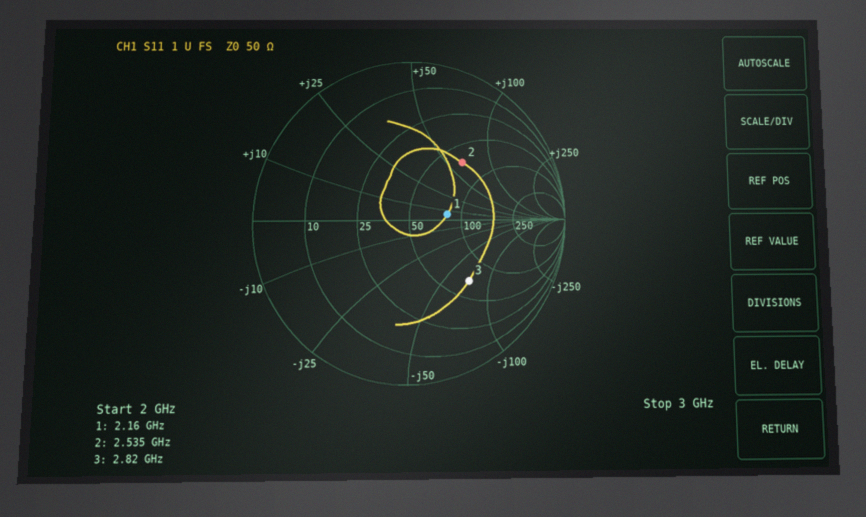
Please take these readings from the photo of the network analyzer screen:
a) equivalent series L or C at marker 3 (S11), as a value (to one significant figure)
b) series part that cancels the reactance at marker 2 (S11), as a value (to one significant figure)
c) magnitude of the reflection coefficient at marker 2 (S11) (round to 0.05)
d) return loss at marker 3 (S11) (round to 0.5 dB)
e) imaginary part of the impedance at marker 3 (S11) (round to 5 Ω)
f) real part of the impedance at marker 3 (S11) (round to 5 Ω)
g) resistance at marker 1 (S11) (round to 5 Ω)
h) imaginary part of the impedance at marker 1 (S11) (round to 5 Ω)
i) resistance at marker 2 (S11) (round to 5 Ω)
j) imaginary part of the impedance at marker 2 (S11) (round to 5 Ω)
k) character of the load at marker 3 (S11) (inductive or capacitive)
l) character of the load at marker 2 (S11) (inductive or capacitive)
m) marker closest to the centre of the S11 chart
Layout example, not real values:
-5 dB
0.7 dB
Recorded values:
800 fF
1.0 pF
0.50
5.5 dB
-70 Ω
70 Ω
80 Ω
+5 Ω
65 Ω
+65 Ω
capacitive
inductive
marker 1
